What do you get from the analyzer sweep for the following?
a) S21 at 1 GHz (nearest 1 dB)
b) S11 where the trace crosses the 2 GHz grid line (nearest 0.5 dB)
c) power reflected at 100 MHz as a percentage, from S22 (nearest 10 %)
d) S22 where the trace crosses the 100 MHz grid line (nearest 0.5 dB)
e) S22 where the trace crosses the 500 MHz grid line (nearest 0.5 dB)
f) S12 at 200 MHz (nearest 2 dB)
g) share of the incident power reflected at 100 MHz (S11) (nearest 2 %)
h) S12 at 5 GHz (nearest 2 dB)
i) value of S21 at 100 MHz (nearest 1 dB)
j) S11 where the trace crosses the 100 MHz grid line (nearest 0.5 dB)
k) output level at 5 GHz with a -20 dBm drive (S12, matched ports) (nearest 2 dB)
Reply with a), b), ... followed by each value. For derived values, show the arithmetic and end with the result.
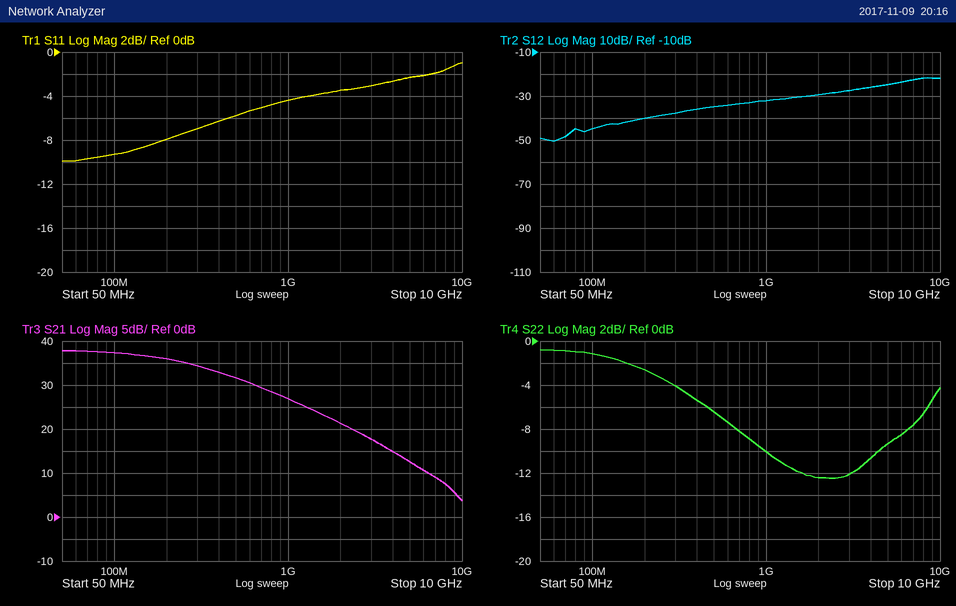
a) 27 dB
b) -3.5 dB
c) 10^(-1/10) ≈ 79.4 %, so 80 % to the nearest 10 %
d) -1.0 dB
e) -6.5 dB
f) -40 dB
g) 10^(-9.5/10) ≈ 11.2 %, so 12 % to the nearest 2 %
h) -24 dB
i) 37 dB
j) -9.5 dB
k) -20 dBm + (-24 dB) = -44 dBm
